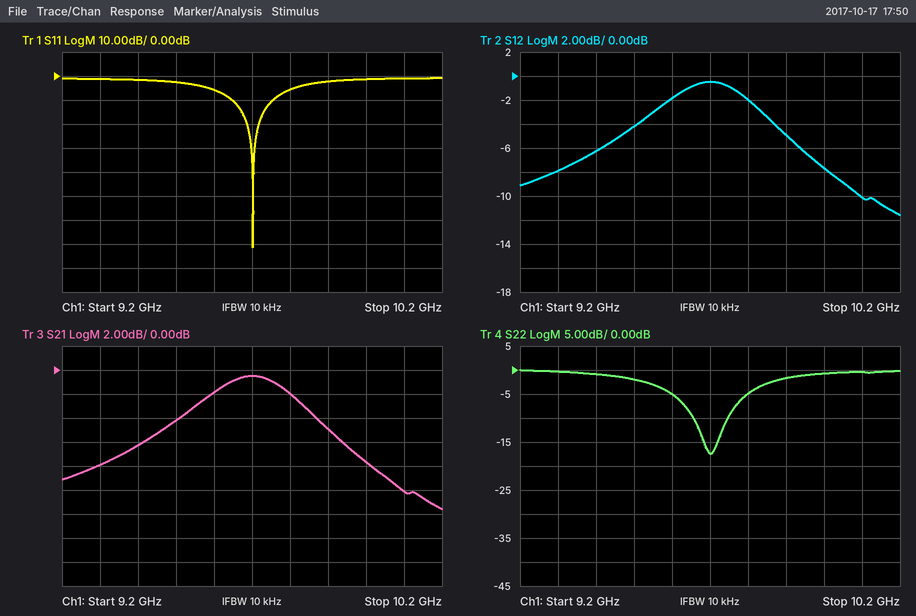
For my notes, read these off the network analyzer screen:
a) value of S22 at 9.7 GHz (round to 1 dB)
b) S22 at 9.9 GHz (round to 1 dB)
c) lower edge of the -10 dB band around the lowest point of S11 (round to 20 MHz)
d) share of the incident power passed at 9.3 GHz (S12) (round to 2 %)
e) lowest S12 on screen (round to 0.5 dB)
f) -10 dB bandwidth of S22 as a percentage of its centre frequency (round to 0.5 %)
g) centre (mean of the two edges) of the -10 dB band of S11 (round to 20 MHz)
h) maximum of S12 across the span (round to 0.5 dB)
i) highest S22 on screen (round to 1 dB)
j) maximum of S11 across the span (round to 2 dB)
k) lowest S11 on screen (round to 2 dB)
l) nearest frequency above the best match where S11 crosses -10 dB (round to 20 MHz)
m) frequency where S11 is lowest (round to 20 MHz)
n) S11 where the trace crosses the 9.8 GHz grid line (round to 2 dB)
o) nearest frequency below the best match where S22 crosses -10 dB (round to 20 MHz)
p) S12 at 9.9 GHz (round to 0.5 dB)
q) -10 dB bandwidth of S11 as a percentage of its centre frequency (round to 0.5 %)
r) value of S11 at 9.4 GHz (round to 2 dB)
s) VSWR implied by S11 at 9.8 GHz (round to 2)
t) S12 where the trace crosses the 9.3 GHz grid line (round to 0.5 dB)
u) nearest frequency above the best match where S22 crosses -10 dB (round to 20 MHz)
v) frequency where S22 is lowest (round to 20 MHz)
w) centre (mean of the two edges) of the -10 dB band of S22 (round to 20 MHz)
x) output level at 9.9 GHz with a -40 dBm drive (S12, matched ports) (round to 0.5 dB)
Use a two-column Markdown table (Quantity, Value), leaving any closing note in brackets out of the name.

| Quantity | Value |
|---|---|
| value of S22 at 9.7 GHz | -17 dB |
| S22 at 9.9 GHz | -2 dB |
| lower edge of the -10 dB band around the lowest point of S11 | 9.64 GHz |
| share of the incident power passed at 9.3 GHz (S12) | 16 % |
| lowest S12 on screen | -11.5 dB |
| -10 dB bandwidth of S22 as a percentage of its centre frequency | 1.0 % |
| centre (mean of the two edges) of the -10 dB band of S11 | 9.70 GHz |
| maximum of S12 across the span | -0.5 dB |
| highest S22 on screen | 0 dB |
| maximum of S11 across the span | 0 dB |
| lowest S11 on screen | -72 dB |
| nearest frequency above the best match where S11 crosses -10 dB | 9.76 GHz |
| frequency where S11 is lowest | 9.70 GHz |
| S11 where the trace crosses the 9.8 GHz grid line | -6 dB |
| nearest frequency below the best match where S22 crosses -10 dB | 9.66 GHz |
| S12 at 9.9 GHz | -5.0 dB |
| -10 dB bandwidth of S11 as a percentage of its centre frequency | 1.0 % |
| value of S11 at 9.4 GHz | -2 dB |
| VSWR implied by S11 at 9.8 GHz | 4 |
| S12 where the trace crosses the 9.3 GHz grid line | -8.0 dB |
| nearest frequency above the best match where S22 crosses -10 dB | 9.74 GHz |
| frequency where S22 is lowest | 9.70 GHz |
| centre (mean of the two edges) of the -10 dB band of S22 | 9.70 GHz |
| output level at 9.9 GHz with a -40 dBm drive (S12, matched ports) | -45.0 dBm |
